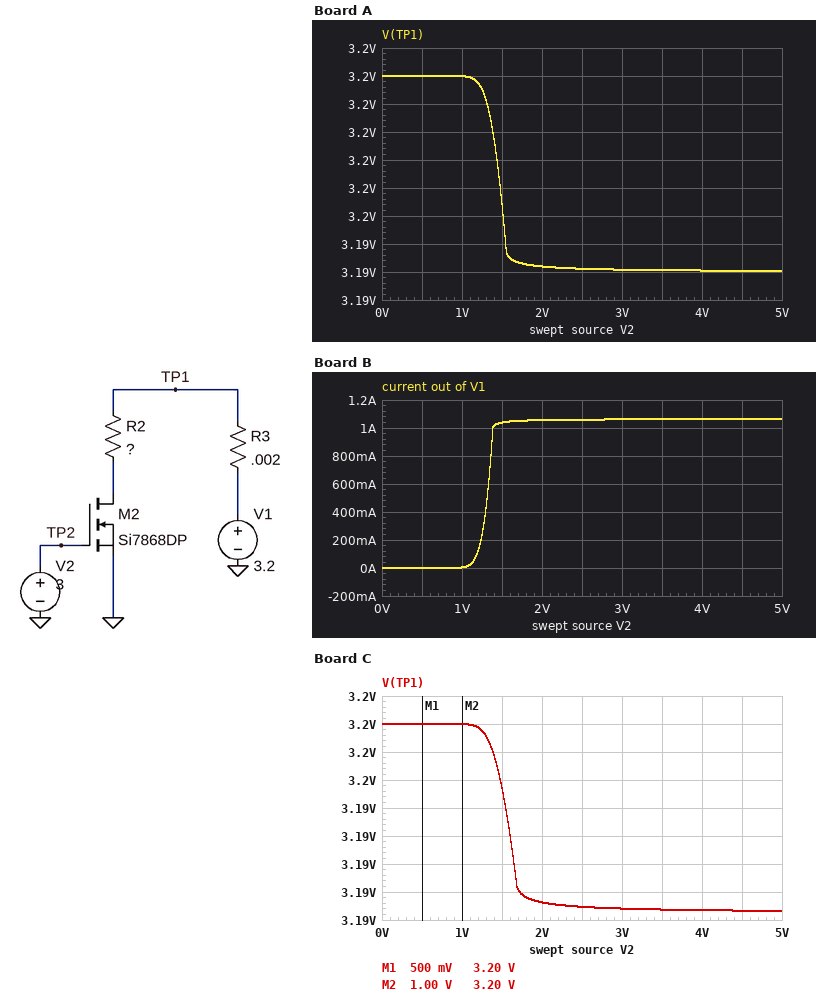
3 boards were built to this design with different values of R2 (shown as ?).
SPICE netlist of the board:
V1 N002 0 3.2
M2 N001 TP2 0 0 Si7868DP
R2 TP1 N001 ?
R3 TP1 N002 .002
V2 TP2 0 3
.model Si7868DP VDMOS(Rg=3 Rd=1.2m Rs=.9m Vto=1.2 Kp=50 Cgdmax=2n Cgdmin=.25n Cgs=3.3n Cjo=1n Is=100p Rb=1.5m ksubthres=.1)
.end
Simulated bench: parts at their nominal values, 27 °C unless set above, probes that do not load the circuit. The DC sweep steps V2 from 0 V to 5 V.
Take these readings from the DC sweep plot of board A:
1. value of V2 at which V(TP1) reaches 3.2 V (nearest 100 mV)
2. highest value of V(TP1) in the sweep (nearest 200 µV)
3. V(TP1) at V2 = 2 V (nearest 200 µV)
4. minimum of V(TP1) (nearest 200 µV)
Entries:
1.5 V
3.2000 V
3.1932 V
3.1930 V
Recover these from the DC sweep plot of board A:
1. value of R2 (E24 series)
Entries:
0.91 Ω
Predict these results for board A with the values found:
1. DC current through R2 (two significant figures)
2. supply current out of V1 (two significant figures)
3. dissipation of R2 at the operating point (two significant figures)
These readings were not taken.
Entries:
3.5 A
3.5 A
11 W
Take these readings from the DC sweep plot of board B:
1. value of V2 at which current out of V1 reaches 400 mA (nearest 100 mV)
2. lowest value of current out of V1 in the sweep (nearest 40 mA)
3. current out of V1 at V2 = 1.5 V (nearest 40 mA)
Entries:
1.3 V
0 A
1.04 A
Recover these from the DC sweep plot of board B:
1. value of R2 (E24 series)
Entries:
3 Ω
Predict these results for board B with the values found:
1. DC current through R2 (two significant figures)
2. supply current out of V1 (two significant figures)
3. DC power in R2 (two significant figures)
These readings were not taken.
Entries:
1.1 A
1.1 A
3.4 W
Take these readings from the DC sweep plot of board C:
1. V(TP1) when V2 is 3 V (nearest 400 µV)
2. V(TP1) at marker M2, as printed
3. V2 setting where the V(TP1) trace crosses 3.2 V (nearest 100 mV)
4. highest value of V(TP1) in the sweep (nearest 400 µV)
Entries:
3.1868 V
3.20 V
1.4 V
3.2000 V
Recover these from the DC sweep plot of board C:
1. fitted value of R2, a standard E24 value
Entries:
0.47 Ω
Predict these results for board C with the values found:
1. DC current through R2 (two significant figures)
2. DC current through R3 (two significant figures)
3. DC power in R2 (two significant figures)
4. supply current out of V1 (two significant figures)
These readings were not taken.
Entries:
6.6 A
6.6 A
20 W
6.6 A
